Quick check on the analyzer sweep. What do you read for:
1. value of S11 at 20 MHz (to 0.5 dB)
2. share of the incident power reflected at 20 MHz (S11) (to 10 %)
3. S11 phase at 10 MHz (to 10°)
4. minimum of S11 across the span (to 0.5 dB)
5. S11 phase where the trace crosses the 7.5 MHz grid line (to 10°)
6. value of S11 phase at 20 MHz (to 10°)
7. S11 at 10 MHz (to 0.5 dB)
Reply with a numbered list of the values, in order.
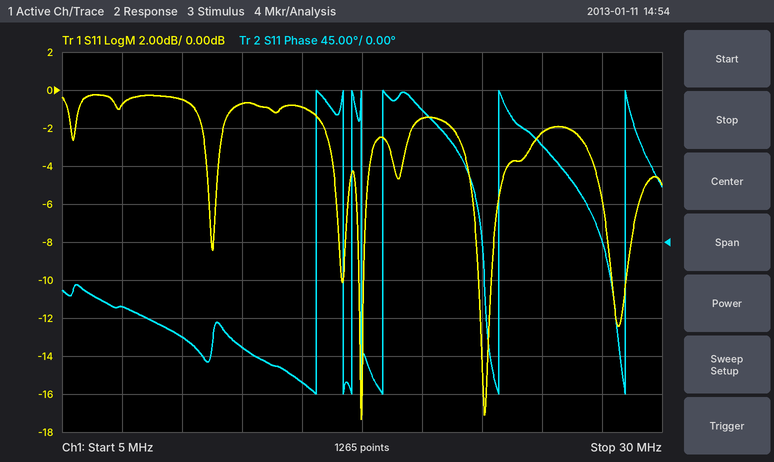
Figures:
1. -1.5 dB
2. 70 %
3. -110°
4. -17.5 dB
5. -80°
6. 160°
7. -0.5 dB
